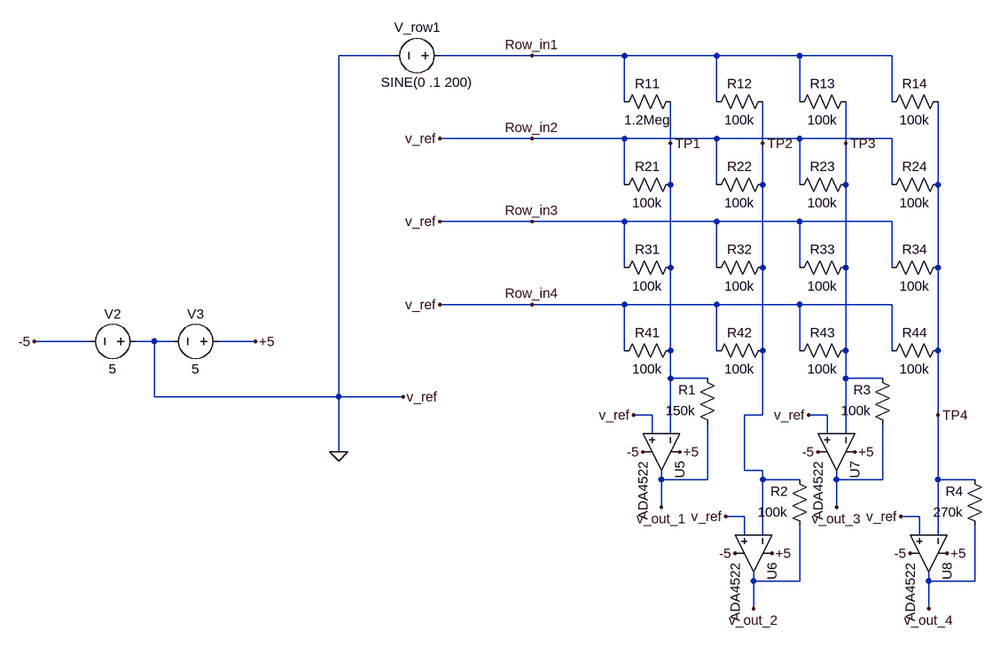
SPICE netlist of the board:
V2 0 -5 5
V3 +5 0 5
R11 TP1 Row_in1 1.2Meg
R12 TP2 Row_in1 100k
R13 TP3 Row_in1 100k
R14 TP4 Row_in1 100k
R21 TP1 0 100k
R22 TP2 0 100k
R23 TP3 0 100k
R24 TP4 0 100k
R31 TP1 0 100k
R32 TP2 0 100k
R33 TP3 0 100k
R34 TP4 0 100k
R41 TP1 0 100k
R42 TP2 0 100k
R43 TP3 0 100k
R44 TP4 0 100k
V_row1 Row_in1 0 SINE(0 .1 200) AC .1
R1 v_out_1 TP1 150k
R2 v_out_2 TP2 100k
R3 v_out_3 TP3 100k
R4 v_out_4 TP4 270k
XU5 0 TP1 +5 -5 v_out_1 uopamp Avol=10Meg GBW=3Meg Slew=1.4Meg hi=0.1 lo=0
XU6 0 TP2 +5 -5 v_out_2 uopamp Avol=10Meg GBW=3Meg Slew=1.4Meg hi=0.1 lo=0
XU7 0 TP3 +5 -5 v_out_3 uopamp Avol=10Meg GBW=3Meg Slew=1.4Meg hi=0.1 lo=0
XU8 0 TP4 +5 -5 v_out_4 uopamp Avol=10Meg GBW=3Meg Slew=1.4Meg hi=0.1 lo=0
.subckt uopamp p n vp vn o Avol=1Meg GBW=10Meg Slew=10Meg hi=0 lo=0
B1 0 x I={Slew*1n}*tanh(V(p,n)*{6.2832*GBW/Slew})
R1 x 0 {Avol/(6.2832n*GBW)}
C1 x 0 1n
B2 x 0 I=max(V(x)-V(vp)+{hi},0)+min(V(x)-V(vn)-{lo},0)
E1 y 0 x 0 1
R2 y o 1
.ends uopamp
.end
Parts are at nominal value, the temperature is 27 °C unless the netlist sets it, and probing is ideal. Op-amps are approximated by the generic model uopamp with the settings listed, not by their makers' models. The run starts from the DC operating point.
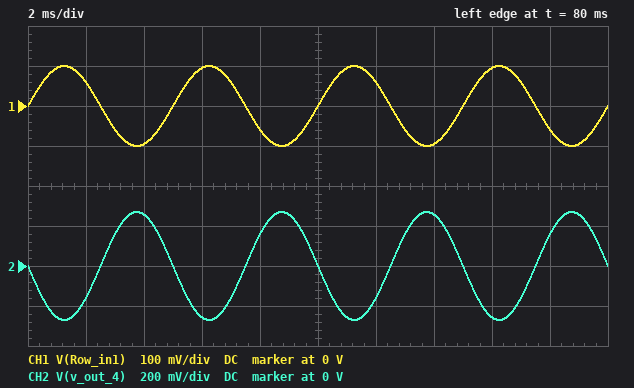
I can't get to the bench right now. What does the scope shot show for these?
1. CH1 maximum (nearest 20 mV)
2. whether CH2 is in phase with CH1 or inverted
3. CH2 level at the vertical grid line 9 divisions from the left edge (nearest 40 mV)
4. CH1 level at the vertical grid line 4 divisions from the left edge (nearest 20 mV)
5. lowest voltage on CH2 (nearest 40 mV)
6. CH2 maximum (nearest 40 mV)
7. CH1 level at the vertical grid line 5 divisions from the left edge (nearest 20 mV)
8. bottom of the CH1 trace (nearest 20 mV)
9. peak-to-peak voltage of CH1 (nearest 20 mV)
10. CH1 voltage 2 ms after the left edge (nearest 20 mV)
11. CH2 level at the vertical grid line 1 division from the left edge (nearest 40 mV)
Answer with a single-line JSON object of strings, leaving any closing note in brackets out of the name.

{"CH1 maximum": "100 mV", "whether CH2 is in phase with CH1 or inverted": "inverted", "CH2 level at the vertical grid line 9 divisions from the left edge": "160 mV", "CH1 level at the vertical grid line 4 divisions from the left edge": "-60 mV", "lowest voltage on CH2": "-280 mV", "CH2 maximum": "280 mV", "CH1 level at the vertical grid line 5 divisions from the left edge": "0 V", "bottom of the CH1 trace": "-100 mV", "peak-to-peak voltage of CH1": "200 mV", "CH1 voltage 2 ms after the left edge": "60 mV", "CH2 level at the vertical grid line 1 division from the left edge": "-160 mV"}
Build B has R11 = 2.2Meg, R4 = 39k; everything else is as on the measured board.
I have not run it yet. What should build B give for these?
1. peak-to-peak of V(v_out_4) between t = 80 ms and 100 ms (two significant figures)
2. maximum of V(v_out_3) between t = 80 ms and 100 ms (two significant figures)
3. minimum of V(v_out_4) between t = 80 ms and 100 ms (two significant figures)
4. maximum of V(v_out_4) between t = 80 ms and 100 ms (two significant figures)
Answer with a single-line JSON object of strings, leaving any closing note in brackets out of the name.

{"peak-to-peak of V(v_out_4) between t = 80 ms and 100 ms": "78 mV", "maximum of V(v_out_3) between t = 80 ms and 100 ms": "100 mV", "minimum of V(v_out_4) between t = 80 ms and 100 ms": "-39 mV", "maximum of V(v_out_4) between t = 80 ms and 100 ms": "39 mV"}
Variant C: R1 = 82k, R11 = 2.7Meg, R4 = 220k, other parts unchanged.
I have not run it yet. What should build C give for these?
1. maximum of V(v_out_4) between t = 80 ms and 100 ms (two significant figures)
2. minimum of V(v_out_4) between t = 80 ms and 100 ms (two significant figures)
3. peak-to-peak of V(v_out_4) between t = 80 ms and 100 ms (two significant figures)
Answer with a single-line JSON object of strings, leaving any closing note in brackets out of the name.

{"maximum of V(v_out_4) between t = 80 ms and 100 ms": "220 mV", "minimum of V(v_out_4) between t = 80 ms and 100 ms": "-220 mV", "peak-to-peak of V(v_out_4) between t = 80 ms and 100 ms": "440 mV"}
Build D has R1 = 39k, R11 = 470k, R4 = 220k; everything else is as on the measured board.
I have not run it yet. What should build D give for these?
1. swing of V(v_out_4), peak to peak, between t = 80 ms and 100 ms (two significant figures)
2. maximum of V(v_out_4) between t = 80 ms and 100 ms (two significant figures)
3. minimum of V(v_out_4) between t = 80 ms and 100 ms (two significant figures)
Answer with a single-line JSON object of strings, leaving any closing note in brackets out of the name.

{"swing of V(v_out_4), peak to peak, between t = 80 ms and 100 ms": "440 mV", "maximum of V(v_out_4) between t = 80 ms and 100 ms": "220 mV", "minimum of V(v_out_4) between t = 80 ms and 100 ms": "-220 mV"}
